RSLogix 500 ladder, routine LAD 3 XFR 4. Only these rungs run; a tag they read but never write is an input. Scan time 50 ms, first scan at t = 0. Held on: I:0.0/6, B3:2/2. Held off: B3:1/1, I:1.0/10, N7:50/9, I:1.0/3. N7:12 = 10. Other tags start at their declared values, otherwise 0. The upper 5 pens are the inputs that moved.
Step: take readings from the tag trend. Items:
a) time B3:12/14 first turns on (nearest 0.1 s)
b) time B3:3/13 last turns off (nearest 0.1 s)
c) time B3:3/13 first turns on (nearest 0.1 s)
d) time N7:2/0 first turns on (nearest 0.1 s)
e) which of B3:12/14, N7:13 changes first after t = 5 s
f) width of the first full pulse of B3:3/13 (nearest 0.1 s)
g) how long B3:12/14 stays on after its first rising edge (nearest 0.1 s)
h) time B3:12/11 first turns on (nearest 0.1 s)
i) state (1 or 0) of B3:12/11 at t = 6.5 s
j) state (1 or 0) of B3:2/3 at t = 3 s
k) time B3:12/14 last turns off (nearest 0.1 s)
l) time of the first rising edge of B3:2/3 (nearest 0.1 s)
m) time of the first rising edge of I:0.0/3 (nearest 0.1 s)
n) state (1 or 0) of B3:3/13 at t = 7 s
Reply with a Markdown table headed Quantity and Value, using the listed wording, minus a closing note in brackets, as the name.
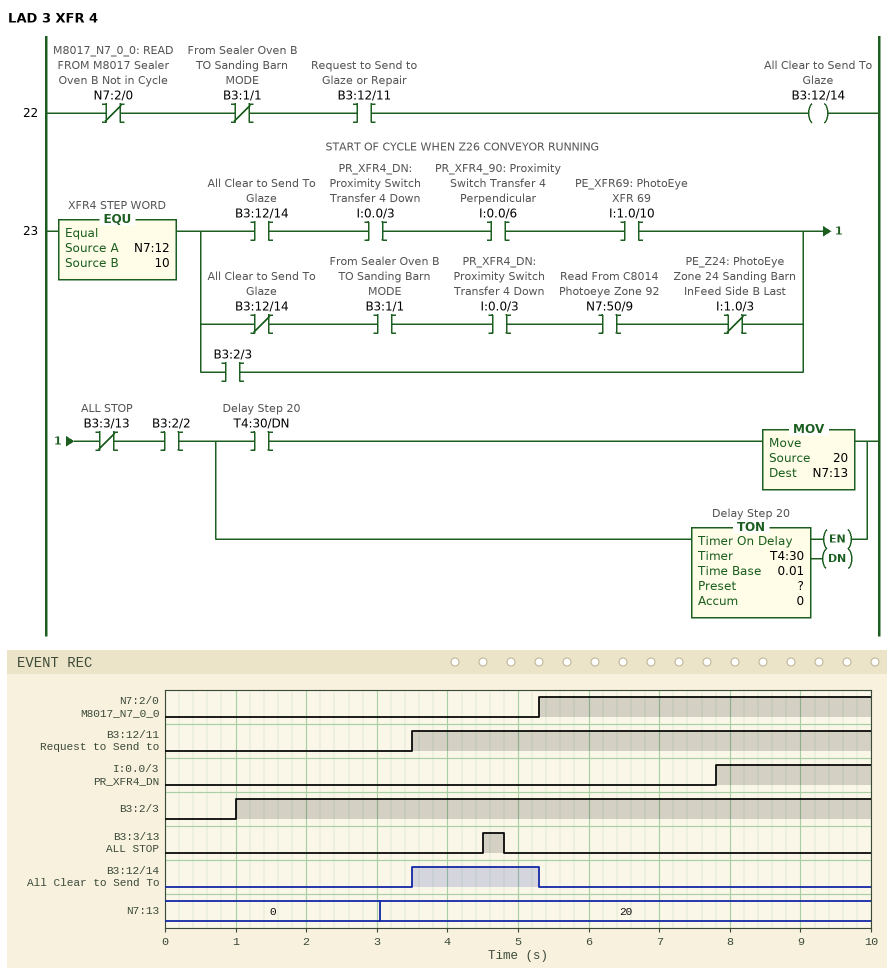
| Quantity | Value |
|---|---|
| time B3:12/14 first turns on | 3.5 s |
| time B3:3/13 last turns off | 4.8 s |
| time B3:3/13 first turns on | 4.5 s |
| time N7:2/0 first turns on | 5.3 s |
| which of B3:12/14, N7:13 changes first after t = 5 s | B3:12/14 |
| width of the first full pulse of B3:3/13 | 0.3 s |
| how long B3:12/14 stays on after its first rising edge | 1.8 s |
| time B3:12/11 first turns on | 3.5 s |
| state (1 or 0) of B3:12/11 at t = 6.5 s | 1 |
| state (1 or 0) of B3:2/3 at t = 3 s | 1 |
| time B3:12/14 last turns off | 5.3 s |
| time of the first rising edge of B3:2/3 | 1.0 s |
| time of the first rising edge of I:0.0/3 | 7.8 s |
| state (1 or 0) of B3:3/13 at t = 7 s | 0 |
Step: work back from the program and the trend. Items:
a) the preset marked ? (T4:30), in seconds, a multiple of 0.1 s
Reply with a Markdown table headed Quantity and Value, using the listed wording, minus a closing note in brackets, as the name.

| Quantity | Value |
|---|---|
| the preset marked ? (T4:30), in seconds, a multiple of 0.1 s | 2.0 s |
